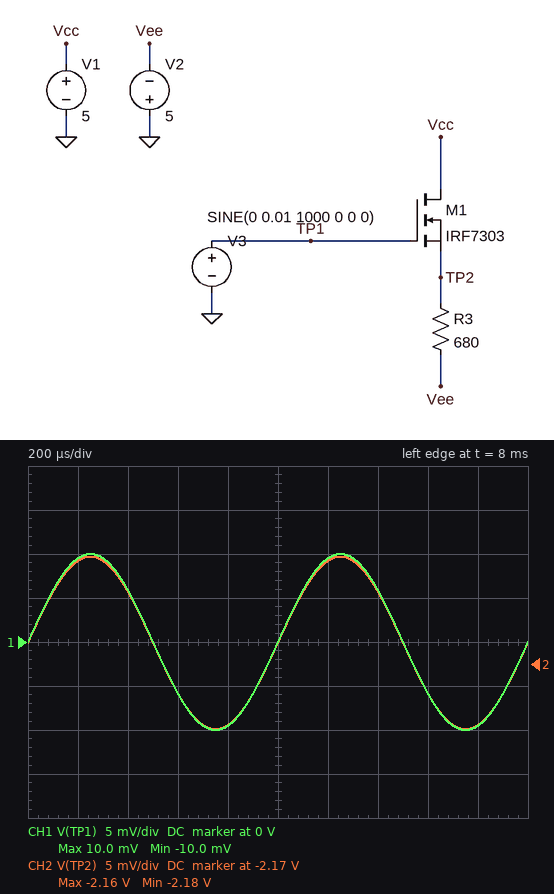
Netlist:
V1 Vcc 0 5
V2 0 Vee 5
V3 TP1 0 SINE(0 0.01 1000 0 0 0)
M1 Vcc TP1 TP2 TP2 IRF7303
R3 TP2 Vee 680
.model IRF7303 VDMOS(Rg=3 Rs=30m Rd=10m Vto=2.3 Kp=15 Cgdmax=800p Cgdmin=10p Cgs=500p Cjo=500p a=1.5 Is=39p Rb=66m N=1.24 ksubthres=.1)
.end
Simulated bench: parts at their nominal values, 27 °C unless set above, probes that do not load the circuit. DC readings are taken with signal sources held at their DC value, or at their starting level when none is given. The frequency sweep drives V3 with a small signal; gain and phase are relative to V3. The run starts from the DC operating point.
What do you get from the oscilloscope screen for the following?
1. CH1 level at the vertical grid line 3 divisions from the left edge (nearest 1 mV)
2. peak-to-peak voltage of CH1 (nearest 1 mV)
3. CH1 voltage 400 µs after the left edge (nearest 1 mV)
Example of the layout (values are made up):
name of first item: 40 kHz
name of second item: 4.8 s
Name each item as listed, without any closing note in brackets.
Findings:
CH1 level at the vertical grid line 3 divisions from the left edge: -6 mV
peak-to-peak voltage of CH1: 20 mV
CH1 voltage 400 µs after the left edge: 6 mV
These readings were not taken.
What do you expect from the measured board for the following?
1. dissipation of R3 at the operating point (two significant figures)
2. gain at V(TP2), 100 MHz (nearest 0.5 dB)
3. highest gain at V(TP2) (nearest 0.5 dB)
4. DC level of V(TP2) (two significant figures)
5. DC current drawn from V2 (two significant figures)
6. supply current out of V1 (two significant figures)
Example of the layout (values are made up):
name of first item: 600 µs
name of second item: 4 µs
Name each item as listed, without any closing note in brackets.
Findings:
dissipation of R3 at the operating point: 12 mW
gain at V(TP2), 100 MHz: -2.5 dB
highest gain at V(TP2): 0 dB
DC level of V(TP2): -2.2 V
DC current drawn from V2: 4.2 mA
supply current out of V1: 4.2 mA
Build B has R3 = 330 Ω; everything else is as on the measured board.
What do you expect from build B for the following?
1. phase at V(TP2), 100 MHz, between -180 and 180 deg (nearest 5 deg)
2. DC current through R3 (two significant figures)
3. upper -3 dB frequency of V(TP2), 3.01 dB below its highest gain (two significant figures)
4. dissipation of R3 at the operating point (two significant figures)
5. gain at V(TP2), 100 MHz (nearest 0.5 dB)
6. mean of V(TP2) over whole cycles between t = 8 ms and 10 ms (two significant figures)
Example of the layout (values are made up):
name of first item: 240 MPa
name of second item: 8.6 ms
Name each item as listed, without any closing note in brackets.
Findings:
phase at V(TP2), 100 MHz, between -180 and 180 deg: -25 deg
DC current through R3: 8.5 mA
upper -3 dB frequency of V(TP2), 3.01 dB below its highest gain: 190 MHz
dissipation of R3 at the operating point: 24 mW
gain at V(TP2), 100 MHz: -2.0 dB
mean of V(TP2) over whole cycles between t = 8 ms and 10 ms: -2.2 V
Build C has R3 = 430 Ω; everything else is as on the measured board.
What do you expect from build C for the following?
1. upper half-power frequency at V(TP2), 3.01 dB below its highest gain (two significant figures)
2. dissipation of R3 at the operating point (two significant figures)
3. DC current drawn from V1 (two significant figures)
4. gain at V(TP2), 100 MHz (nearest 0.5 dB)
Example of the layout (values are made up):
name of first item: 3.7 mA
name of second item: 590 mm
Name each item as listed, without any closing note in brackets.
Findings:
upper half-power frequency at V(TP2), 3.01 dB below its highest gain: 180 MHz
dissipation of R3 at the operating point: 18 mW
DC current drawn from V1: 6.5 mA
gain at V(TP2), 100 MHz: -2.0 dB
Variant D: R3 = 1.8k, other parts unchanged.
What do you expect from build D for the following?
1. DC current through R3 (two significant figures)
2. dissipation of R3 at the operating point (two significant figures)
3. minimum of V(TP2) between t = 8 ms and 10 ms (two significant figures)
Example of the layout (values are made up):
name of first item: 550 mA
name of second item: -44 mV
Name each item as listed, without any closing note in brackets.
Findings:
DC current through R3: 1.6 mA
dissipation of R3 at the operating point: 4.6 mW
minimum of V(TP2) between t = 8 ms and 10 ms: -2.1 V
